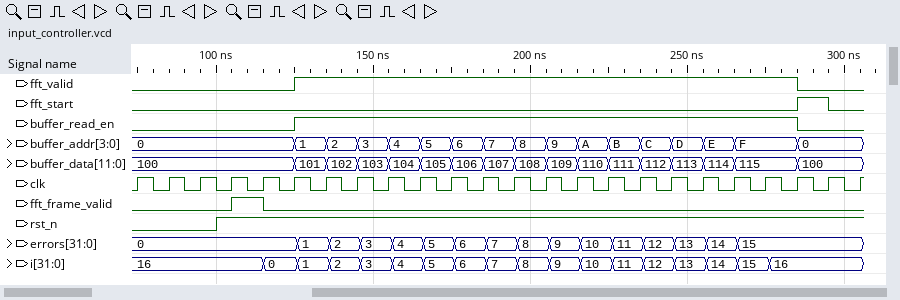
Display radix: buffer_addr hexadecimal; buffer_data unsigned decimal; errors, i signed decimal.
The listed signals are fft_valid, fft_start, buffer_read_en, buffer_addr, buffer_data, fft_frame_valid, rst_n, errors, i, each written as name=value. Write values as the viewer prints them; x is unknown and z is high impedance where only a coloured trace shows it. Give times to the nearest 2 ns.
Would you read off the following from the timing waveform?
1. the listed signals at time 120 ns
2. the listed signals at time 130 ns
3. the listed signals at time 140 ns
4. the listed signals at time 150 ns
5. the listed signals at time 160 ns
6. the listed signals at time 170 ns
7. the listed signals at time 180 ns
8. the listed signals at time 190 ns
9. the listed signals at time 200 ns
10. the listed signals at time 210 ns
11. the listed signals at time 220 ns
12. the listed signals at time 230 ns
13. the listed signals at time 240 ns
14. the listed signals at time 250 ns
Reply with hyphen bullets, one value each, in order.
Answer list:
- fft_valid=0, fft_start=0, buffer_read_en=0, buffer_addr=0, buffer_data=100, fft_frame_valid=0, rst_n=1, errors=0, i=0
- fft_valid=1, fft_start=0, buffer_read_en=1, buffer_addr=1, buffer_data=101, fft_frame_valid=0, rst_n=1, errors=1, i=1
- fft_valid=1, fft_start=0, buffer_read_en=1, buffer_addr=2, buffer_data=102, fft_frame_valid=0, rst_n=1, errors=2, i=2
- fft_valid=1, fft_start=0, buffer_read_en=1, buffer_addr=3, buffer_data=103, fft_frame_valid=0, rst_n=1, errors=3, i=3
- fft_valid=1, fft_start=0, buffer_read_en=1, buffer_addr=4, buffer_data=104, fft_frame_valid=0, rst_n=1, errors=4, i=4
- fft_valid=1, fft_start=0, buffer_read_en=1, buffer_addr=5, buffer_data=105, fft_frame_valid=0, rst_n=1, errors=5, i=5
- fft_valid=1, fft_start=0, buffer_read_en=1, buffer_addr=6, buffer_data=106, fft_frame_valid=0, rst_n=1, errors=6, i=6
- fft_valid=1, fft_start=0, buffer_read_en=1, buffer_addr=7, buffer_data=107, fft_frame_valid=0, rst_n=1, errors=7, i=7
- fft_valid=1, fft_start=0, buffer_read_en=1, buffer_addr=8, buffer_data=108, fft_frame_valid=0, rst_n=1, errors=8, i=8
- fft_valid=1, fft_start=0, buffer_read_en=1, buffer_addr=9, buffer_data=109, fft_frame_valid=0, rst_n=1, errors=9, i=9
- fft_valid=1, fft_start=0, buffer_read_en=1, buffer_addr=A, buffer_data=110, fft_frame_valid=0, rst_n=1, errors=10, i=10
- fft_valid=1, fft_start=0, buffer_read_en=1, buffer_addr=B, buffer_data=111, fft_frame_valid=0, rst_n=1, errors=11, i=11
- fft_valid=1, fft_start=0, buffer_read_en=1, buffer_addr=C, buffer_data=112, fft_frame_valid=0, rst_n=1, errors=12, i=12
- fft_valid=1, fft_start=0, buffer_read_en=1, buffer_addr=D, buffer_data=113, fft_frame_valid=0, rst_n=1, errors=13, i=13
